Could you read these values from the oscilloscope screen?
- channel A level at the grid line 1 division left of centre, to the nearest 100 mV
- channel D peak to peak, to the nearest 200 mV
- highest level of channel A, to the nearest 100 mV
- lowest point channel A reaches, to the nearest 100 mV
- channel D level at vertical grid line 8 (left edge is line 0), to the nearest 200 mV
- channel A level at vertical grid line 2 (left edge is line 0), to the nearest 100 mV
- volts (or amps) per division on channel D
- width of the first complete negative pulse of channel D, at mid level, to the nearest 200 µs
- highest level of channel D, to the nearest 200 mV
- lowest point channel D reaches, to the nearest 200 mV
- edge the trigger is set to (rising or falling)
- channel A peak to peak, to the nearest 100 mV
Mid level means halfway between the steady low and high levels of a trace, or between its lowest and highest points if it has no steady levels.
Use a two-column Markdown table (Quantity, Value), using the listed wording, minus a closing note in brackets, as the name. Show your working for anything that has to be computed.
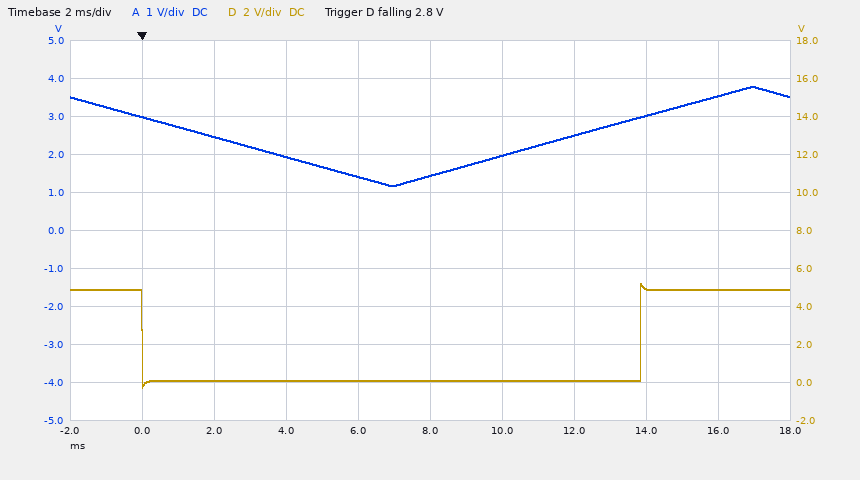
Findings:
| Quantity | Value |
|---|---|
| channel A level at the grid line 1 division left of centre, to the nearest 100 mV | 1.4 V |
| channel D peak to peak, to the nearest 200 mV | 5.2 V − (-200 mV) = 5.4 V |
| highest level of channel A, to the nearest 100 mV | 3.8 V |
| lowest point channel A reaches, to the nearest 100 mV | 1.2 V |
| channel D level at vertical grid line 8 (left edge is line 0), to the nearest 200 mV | 5.0 V |
| channel A level at vertical grid line 2 (left edge is line 0), to the nearest 100 mV | 2.5 V |
| volts (or amps) per division on channel D | 2 V |
| width of the first complete negative pulse of channel D, at mid level, to the nearest 200 µs | 13.8 ms |
| highest level of channel D, to the nearest 200 mV | 5.2 V |
| lowest point channel D reaches, to the nearest 200 mV | -200 mV |
| edge the trigger is set to | falling |
| channel A peak to peak, to the nearest 100 mV | 3.8 V − (1.2 V) = 2.6 V |
